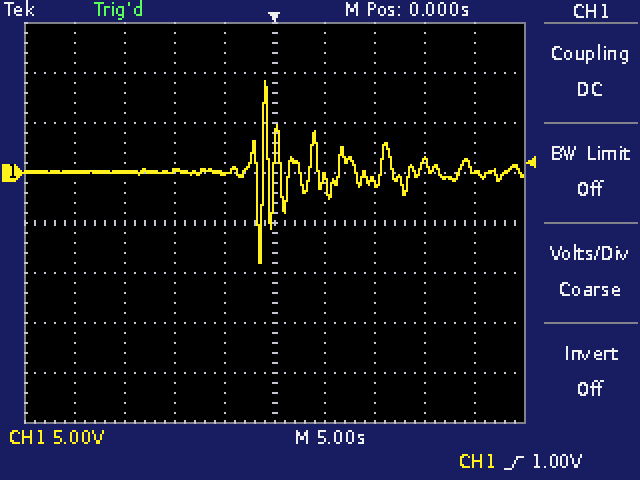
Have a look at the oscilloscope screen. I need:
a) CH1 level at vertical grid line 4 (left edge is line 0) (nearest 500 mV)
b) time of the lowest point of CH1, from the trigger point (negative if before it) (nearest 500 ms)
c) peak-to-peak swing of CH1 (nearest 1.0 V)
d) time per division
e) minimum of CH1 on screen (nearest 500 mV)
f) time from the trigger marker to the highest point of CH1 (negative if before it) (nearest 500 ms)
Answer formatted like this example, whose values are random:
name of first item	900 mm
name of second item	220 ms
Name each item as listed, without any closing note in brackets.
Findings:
CH1 level at vertical grid line 4 (left edge is line 0)	0.0 V
time of the lowest point of CH1, from the trigger point (negative if before it)	-1.5 s
peak-to-peak swing of CH1	18.0 V
time per division	5 s
minimum of CH1 on screen	-9.0 V
time from the trigger marker to the highest point of CH1 (negative if before it)	-1.0 s
